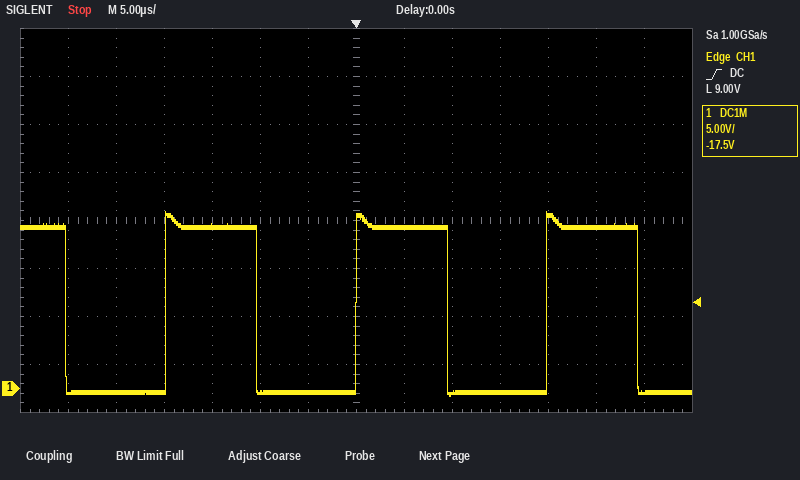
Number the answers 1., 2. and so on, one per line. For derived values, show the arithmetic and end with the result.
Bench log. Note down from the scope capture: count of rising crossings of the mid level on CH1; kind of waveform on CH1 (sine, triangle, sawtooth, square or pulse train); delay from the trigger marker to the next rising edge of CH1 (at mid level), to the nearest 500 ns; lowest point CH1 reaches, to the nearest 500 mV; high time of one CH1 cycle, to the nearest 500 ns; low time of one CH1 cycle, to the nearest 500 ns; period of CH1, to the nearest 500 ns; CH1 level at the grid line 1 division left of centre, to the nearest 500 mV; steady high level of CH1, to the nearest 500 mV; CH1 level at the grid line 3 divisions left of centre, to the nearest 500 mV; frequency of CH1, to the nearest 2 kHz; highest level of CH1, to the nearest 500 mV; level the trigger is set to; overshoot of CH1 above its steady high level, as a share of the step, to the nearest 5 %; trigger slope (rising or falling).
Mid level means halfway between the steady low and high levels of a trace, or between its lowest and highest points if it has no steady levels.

1. 3
2. square
3. 20.0 µs
4. -1.0 V
5. 9.5 µs
6. 10.5 µs
7. 20.0 µs
8. -500 mV
9. 17.0 V
10. 17.0 V
11. 1 / 20.0 µs ≈ 50 kHz
12. 18.5 V
13. 9.00 V
14. 10 %
15. rising
